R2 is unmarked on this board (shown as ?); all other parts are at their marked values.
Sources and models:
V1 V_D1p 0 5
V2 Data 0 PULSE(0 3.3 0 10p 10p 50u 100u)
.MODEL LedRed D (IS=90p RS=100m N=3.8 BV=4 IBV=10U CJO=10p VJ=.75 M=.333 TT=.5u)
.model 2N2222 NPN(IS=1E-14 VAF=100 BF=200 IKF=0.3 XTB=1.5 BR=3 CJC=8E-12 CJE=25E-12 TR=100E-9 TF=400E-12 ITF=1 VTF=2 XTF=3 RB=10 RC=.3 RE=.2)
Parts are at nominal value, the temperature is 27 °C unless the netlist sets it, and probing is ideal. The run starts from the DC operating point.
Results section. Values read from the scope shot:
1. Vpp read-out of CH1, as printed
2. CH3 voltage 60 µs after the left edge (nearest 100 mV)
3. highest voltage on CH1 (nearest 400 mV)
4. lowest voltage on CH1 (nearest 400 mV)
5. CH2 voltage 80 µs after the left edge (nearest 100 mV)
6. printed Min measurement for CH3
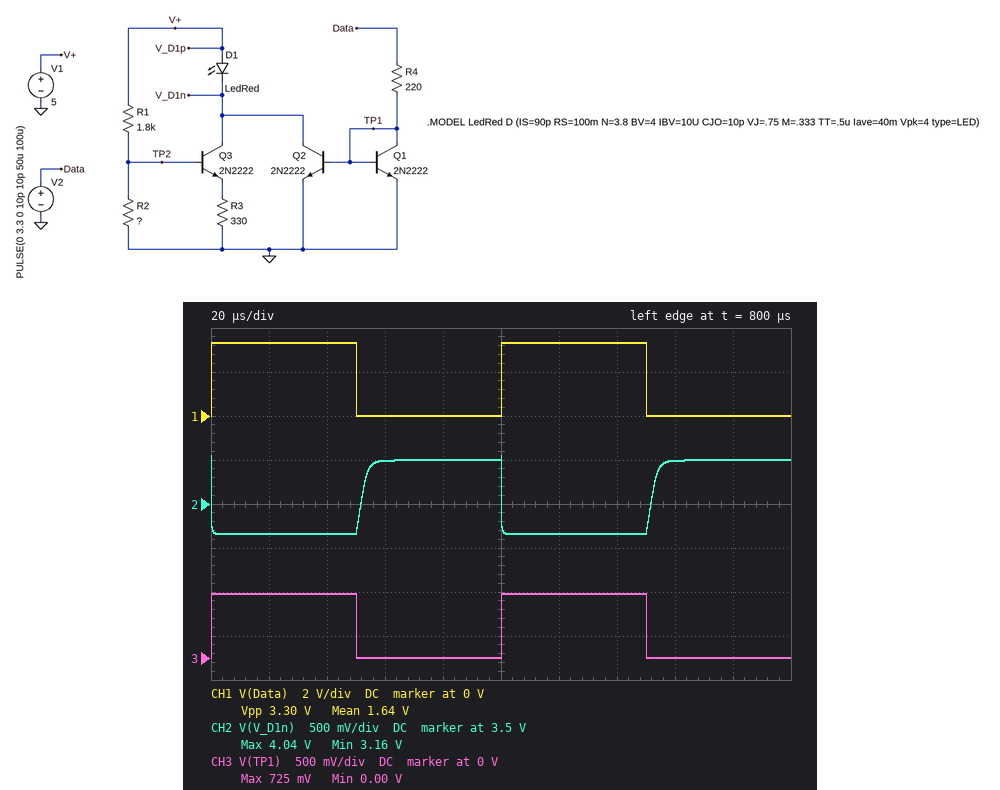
3.30 V
0 V
3.2 V
0 V
4.0 V
0.00 V
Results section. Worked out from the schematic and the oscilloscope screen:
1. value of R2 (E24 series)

200 Ω
